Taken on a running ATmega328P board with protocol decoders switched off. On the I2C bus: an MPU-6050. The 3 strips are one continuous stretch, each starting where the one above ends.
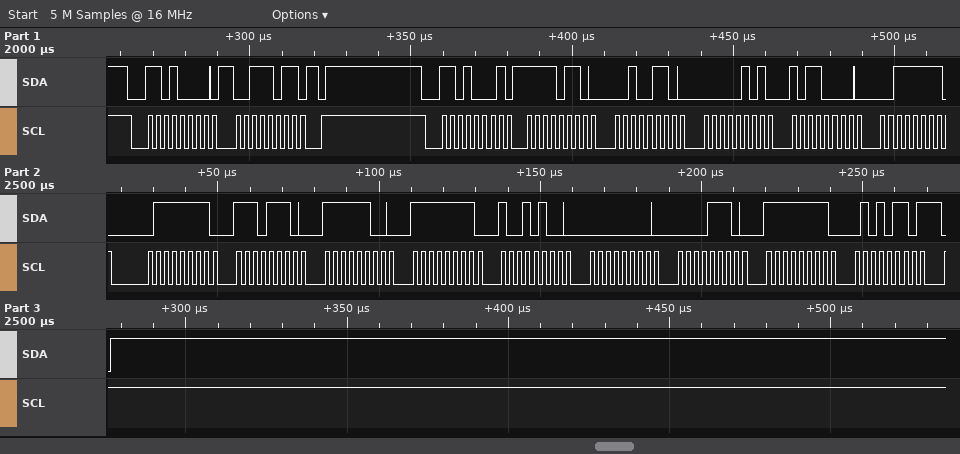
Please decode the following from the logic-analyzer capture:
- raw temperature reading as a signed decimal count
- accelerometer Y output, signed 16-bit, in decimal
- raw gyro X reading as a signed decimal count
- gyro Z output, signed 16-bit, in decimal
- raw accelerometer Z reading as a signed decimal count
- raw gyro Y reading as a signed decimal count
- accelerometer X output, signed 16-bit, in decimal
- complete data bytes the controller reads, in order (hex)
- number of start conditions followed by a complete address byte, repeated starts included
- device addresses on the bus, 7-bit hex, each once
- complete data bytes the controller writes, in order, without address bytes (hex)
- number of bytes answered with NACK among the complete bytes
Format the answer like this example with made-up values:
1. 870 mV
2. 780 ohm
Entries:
1. -4356
2. 1456
3. -108
4. -170
5. 16255
6. 14
7. -2522
8. F6 26 05 B0 3F 7F EE FC FF 94 00 0E FF 56
9. 2
10. 0x68
11. 3B
12. 1
